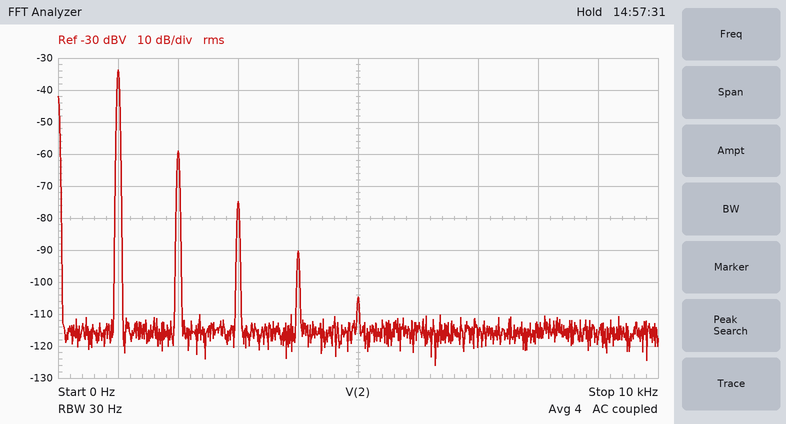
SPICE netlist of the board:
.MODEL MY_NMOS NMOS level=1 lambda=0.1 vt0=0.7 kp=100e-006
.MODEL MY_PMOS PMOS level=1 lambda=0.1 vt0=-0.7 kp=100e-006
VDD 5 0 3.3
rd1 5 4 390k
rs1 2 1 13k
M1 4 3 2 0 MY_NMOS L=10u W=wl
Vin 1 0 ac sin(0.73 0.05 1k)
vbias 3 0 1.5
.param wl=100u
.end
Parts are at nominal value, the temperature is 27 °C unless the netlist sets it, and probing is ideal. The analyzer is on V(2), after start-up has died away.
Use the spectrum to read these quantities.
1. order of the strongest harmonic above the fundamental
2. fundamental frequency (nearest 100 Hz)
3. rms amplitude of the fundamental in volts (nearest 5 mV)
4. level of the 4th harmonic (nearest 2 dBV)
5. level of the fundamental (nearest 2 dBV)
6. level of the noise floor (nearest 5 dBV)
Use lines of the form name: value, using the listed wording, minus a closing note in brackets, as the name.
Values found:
order of the strongest harmonic above the fundamental: 2
fundamental frequency: 1.0 kHz
rms amplitude of the fundamental in volts: 20 mV
level of the 4th harmonic: -90 dBV
level of the fundamental: -34 dBV
level of the noise floor: -115 dBV
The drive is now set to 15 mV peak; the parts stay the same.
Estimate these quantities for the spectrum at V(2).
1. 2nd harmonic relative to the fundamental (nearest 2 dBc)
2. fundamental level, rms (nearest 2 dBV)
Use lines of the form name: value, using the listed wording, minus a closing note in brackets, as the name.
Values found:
2nd harmonic relative to the fundamental: -36 dBc
fundamental level, rms: -44 dBV
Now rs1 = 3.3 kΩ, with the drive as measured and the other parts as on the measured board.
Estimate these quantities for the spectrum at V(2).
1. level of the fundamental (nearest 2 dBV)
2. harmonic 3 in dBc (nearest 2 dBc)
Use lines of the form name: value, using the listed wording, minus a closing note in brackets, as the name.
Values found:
level of the fundamental: -30 dBV
harmonic 3 in dBc: -50 dBc
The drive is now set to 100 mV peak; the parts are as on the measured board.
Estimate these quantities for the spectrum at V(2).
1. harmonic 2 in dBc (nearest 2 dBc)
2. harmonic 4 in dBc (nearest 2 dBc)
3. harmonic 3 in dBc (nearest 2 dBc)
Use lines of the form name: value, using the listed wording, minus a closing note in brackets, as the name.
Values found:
harmonic 2 in dBc: -18 dBc
harmonic 4 in dBc: -54 dBc
harmonic 3 in dBc: -30 dBc
